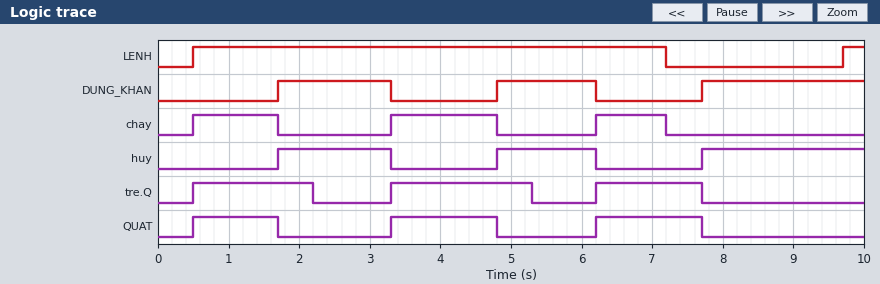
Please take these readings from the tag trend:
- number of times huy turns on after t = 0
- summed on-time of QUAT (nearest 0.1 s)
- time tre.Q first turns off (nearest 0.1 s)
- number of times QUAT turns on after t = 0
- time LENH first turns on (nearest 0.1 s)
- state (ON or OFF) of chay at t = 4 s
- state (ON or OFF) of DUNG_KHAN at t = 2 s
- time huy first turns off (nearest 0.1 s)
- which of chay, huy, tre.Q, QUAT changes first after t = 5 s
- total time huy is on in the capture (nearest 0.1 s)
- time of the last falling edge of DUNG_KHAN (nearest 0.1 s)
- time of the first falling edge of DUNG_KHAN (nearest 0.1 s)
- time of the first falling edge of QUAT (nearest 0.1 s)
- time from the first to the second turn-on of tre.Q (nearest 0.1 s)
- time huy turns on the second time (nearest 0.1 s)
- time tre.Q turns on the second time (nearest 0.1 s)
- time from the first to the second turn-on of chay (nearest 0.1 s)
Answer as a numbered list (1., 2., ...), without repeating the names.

1. 3
2. 4.2 s
3. 2.2 s
4. 3
5. 0.5 s
6. ON
7. ON
8. 3.3 s
9. tre.Q
10. 5.3 s
11. 6.2 s
12. 3.3 s
13. 1.7 s
14. 2.8 s
15. 4.8 s
16. 3.3 s
17. 2.8 s
